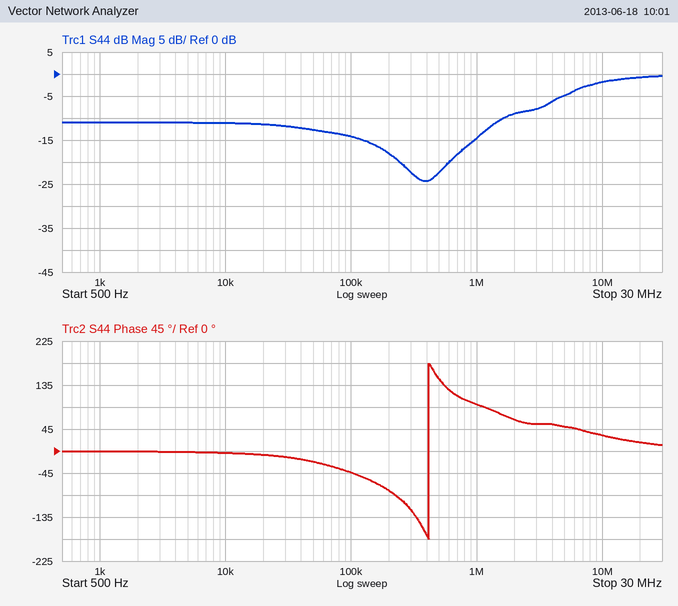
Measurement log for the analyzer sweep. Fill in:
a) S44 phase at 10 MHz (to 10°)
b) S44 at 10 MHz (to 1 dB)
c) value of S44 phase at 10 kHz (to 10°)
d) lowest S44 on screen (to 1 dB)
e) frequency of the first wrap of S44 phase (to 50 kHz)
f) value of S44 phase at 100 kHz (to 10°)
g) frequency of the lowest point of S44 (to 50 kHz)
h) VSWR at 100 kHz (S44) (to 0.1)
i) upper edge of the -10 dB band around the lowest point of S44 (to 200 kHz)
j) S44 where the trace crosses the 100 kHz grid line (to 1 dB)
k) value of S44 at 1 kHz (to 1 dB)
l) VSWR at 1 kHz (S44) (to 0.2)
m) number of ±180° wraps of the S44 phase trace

30°
-2 dB
0°
-24 dB
400 kHz
-40°
400 kHz
1.5
1.6 MHz
-14 dB
-11 dB
1.8
1
